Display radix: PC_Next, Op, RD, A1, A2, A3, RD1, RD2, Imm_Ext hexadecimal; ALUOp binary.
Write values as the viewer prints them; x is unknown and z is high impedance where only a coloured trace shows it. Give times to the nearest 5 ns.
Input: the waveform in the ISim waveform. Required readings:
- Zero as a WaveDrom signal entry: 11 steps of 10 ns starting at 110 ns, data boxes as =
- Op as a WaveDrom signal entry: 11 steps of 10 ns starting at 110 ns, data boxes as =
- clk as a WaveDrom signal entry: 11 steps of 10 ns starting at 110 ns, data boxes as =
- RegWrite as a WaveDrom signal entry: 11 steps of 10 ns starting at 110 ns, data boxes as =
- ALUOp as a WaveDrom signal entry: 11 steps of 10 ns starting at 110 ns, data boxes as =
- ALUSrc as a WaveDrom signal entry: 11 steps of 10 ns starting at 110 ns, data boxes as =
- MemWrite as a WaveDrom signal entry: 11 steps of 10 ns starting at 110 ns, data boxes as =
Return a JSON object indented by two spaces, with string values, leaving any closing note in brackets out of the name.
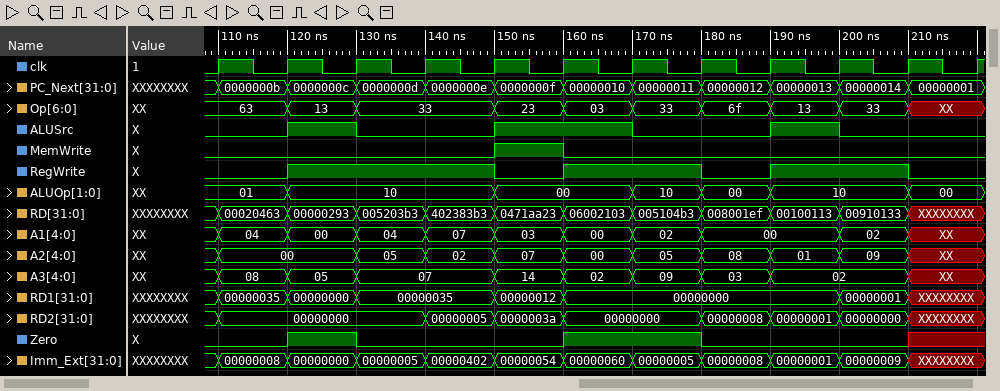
{
  "Zero as a WaveDrom signal entry: 11 steps of 10 ns starting at 110 ns, data boxes as =": "{name: 'Zero', wave: '010..1.0..x'}",
  "Op as a WaveDrom signal entry: 11 steps of 10 ns starting at 110 ns, data boxes as =": "{name: 'Op', wave: '===.======x', data: '63 13 33 23 03 33 6f 13 33'}",
  "clk as a WaveDrom signal entry: 11 steps of 10 ns starting at 110 ns, data boxes as =": "{name: 'clk', wave: 'p..........'}",
  "RegWrite as a WaveDrom signal entry: 11 steps of 10 ns starting at 110 ns, data boxes as =": "{name: 'RegWrite', wave: '01..01.01.0'}",
  "ALUOp as a WaveDrom signal entry: 11 steps of 10 ns starting at 110 ns, data boxes as =": "{name: 'ALUOp', wave: '==..=.===.=', data: '01 10 00 10 00 10 00'}",
  "ALUSrc as a WaveDrom signal entry: 11 steps of 10 ns starting at 110 ns, data boxes as =": "{name: 'ALUSrc', wave: '010.1.0.10.'}",
  "MemWrite as a WaveDrom signal entry: 11 steps of 10 ns starting at 110 ns, data boxes as =": "{name: 'MemWrite', wave: '0...10.....'}"
}
